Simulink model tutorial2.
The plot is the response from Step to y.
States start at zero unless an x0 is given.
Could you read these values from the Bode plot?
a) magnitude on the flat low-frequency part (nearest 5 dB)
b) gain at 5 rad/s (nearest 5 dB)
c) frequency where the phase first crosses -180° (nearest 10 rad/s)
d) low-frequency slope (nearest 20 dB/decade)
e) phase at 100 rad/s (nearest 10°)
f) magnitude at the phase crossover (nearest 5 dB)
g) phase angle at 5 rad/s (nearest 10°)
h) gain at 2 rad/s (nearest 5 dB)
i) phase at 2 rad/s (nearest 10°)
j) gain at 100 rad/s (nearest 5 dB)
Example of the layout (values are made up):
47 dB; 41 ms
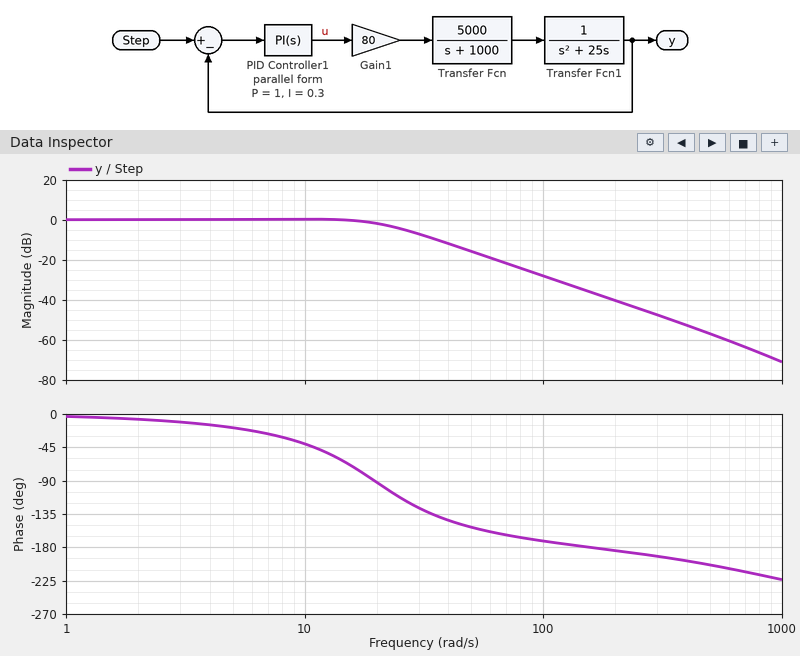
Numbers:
0 dB; 0 dB; 160 rad/s; 0 dB/decade; -170°; -35 dB; -20°; 0 dB; -10°; -30 dB
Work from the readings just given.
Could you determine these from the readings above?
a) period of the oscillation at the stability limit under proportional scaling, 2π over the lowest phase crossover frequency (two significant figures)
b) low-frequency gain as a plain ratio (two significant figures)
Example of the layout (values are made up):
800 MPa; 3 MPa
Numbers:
0.039 s; 1.0
